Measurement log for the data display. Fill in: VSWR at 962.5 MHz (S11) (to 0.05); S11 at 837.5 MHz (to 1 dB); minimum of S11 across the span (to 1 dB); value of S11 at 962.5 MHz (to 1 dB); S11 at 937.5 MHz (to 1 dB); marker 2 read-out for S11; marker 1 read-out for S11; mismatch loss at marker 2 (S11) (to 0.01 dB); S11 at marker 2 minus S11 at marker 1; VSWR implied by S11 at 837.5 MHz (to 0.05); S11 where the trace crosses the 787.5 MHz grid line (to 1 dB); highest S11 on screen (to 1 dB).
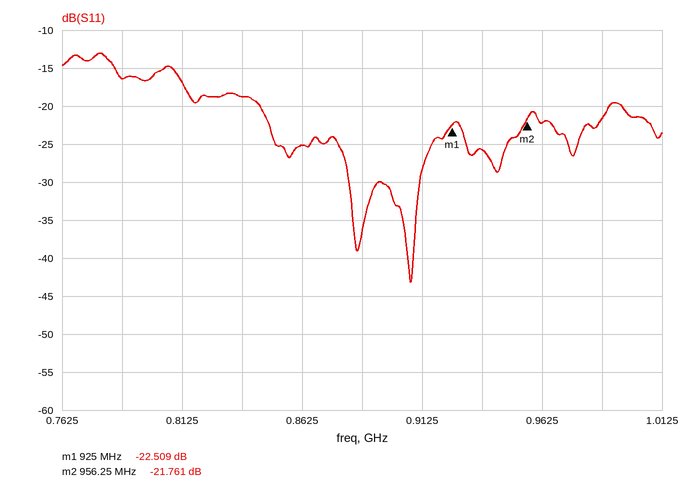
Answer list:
1.15
-19 dB
-43 dB
-22 dB
-26 dB
-21.761 dB
-22.509 dB
0.03 dB
0.748 dB
1.25
-16 dB
-13 dB
